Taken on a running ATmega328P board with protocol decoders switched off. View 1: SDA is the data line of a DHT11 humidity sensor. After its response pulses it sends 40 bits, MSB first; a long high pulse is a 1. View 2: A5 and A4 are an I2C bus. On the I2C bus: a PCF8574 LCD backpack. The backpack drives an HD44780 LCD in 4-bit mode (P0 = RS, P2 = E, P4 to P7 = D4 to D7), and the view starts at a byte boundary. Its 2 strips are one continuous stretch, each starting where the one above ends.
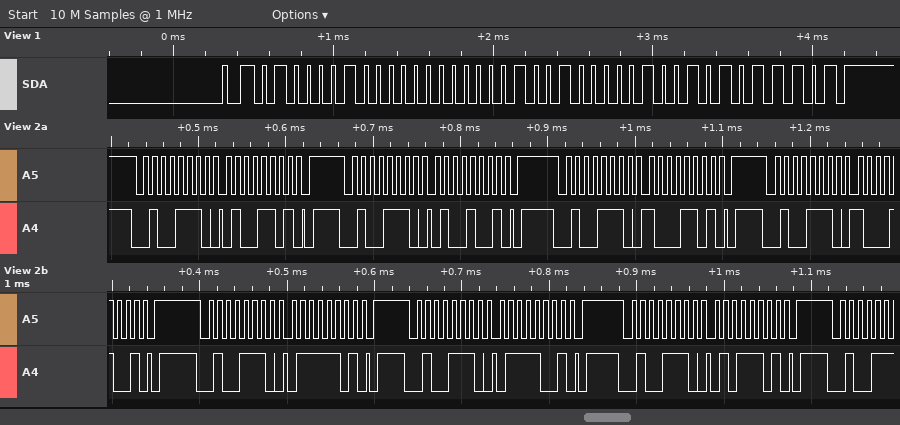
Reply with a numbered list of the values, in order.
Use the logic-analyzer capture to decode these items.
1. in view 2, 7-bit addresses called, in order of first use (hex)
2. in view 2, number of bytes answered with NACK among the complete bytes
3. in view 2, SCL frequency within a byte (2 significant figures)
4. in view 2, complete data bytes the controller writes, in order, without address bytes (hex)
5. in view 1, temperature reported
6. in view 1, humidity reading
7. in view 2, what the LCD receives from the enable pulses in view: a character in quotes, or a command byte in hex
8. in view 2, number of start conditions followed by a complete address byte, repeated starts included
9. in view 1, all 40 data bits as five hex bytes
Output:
1. 0x27
2. 0
3. 100 kHz
4. 4D 49 8D 89 7D 79 5D
5. 18.9 °C
6. 66 %
7. 'H'
8. 7
9. 42 00 12 09 5D
